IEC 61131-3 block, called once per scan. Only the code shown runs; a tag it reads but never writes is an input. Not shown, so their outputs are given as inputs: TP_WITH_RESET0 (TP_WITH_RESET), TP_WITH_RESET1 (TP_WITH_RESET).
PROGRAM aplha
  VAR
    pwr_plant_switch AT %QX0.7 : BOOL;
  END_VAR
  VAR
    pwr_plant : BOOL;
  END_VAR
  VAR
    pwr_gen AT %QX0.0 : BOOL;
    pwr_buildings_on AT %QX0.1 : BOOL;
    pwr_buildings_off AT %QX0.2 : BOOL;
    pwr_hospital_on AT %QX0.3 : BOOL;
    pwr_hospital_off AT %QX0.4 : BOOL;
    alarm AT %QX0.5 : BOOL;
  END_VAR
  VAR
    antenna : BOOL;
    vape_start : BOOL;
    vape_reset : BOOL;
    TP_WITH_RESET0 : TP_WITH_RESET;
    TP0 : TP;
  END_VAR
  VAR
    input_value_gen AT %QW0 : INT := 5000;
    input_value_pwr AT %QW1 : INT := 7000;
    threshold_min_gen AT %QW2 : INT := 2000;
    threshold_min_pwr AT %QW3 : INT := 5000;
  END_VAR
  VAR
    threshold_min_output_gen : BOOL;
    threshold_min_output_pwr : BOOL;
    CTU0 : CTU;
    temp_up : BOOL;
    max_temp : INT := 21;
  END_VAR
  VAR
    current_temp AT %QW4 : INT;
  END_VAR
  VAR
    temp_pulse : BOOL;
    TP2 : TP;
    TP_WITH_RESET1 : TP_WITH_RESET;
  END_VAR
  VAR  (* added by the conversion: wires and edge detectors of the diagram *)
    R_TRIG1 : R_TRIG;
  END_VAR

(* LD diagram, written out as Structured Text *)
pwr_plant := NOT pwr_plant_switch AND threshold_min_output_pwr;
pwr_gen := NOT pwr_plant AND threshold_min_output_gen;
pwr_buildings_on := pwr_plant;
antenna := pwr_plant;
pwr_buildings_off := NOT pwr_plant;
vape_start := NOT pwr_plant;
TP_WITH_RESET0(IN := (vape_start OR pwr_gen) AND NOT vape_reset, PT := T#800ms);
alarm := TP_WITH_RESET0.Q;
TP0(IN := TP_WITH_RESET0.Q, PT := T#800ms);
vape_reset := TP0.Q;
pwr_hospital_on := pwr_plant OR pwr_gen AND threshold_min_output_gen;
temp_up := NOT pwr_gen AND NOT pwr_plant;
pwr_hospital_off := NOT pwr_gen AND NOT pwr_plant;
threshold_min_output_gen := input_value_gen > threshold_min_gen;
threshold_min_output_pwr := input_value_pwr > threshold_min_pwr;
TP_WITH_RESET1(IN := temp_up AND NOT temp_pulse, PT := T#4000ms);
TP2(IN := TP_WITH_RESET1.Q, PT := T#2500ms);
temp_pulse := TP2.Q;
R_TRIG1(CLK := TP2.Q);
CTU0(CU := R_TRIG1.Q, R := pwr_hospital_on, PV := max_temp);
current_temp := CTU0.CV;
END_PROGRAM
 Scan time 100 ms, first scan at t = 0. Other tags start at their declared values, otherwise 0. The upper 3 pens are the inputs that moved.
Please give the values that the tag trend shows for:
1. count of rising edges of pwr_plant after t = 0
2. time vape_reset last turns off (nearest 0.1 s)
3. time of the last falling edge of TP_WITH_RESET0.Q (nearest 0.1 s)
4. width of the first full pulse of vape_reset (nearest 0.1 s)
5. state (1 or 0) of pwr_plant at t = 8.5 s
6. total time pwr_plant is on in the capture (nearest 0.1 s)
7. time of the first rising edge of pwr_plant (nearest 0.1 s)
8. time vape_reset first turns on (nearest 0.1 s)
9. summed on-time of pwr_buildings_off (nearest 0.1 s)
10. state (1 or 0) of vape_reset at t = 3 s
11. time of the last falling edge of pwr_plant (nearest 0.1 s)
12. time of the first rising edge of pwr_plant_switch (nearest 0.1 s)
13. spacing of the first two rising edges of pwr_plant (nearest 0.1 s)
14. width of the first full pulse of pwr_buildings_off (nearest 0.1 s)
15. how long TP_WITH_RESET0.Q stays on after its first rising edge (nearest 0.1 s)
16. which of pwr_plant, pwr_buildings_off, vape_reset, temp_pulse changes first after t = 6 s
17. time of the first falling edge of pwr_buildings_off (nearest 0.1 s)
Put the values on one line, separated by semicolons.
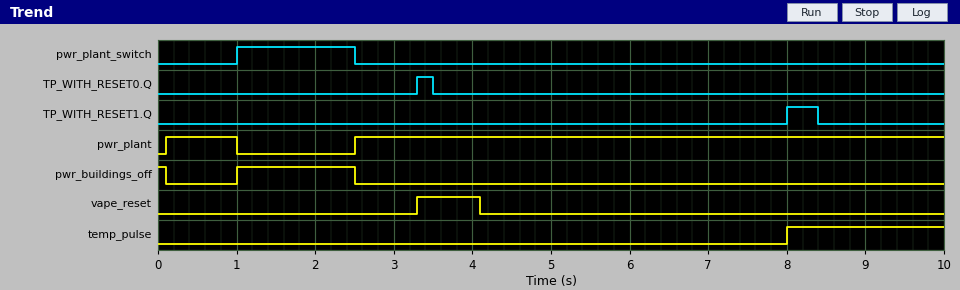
2; 4.1 s; 3.5 s; 0.8 s; 1; 8.4 s; 0.1 s; 3.3 s; 1.6 s; 0; 1.0 s; 1.0 s; 2.4 s; 1.5 s; 0.2 s; temp_pulse; 0.1 s
